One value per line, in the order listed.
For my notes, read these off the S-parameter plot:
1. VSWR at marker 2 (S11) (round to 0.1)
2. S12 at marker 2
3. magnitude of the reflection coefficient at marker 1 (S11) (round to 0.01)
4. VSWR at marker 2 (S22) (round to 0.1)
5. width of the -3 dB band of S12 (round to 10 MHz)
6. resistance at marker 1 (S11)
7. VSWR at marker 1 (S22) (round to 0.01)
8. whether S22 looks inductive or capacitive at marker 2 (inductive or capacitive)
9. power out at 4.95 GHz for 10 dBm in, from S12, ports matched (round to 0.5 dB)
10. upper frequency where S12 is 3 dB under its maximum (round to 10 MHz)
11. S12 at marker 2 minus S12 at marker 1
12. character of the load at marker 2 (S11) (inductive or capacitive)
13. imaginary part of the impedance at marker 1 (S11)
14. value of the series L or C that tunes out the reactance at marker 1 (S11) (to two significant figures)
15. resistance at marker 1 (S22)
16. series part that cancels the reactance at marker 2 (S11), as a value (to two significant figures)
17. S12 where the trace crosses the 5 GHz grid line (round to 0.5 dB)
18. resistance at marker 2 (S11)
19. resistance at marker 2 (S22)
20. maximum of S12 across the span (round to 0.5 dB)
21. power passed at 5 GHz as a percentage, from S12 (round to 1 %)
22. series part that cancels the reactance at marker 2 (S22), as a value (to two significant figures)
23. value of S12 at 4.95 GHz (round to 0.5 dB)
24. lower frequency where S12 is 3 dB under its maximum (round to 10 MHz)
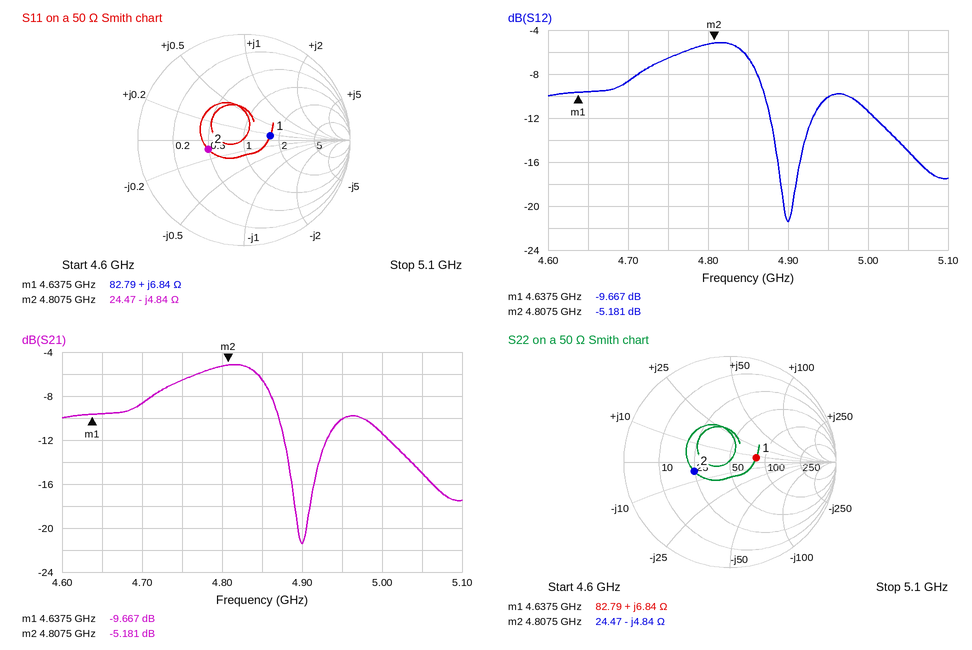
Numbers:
2.1
-5.181 dB
0.25
2.1
150 MHz
82.79 Ω
1.67
capacitive
0.0 dBm
4.86 GHz
4.486 dB
capacitive
+6.84 Ω
5.0 pF
82.79 Ω
160 pH
-11.5 dB
24.47 Ω
24.47 Ω
-5.0 dB
7 %
160 pH
-10.0 dB
4.71 GHz
